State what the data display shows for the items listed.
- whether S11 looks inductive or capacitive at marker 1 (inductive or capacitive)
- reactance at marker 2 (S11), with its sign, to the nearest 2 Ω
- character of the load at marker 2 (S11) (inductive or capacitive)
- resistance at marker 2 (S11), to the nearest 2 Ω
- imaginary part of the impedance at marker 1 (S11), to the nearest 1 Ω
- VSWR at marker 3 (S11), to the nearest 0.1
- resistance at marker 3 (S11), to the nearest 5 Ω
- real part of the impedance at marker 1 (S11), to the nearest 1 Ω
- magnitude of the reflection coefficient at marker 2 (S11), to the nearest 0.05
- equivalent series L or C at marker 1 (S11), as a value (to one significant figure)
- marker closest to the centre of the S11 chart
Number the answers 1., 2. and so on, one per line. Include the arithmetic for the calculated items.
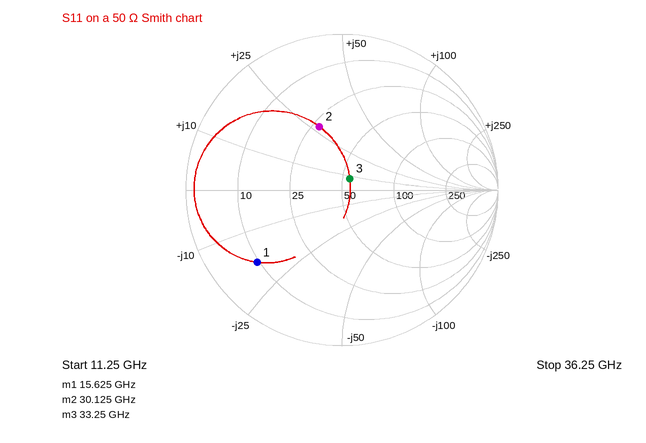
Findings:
1. capacitive
2. +28 Ω
3. inductive
4. 28 Ω
5. -18 Ω
6. 1.2
7. 55 Ω
8. 9 Ω
9. 0.45
10. C = 1/(2π × 15.625 GHz × 18 Ω) ≈ 566 fF, so 600 fF to one significant figure
11. marker 3
